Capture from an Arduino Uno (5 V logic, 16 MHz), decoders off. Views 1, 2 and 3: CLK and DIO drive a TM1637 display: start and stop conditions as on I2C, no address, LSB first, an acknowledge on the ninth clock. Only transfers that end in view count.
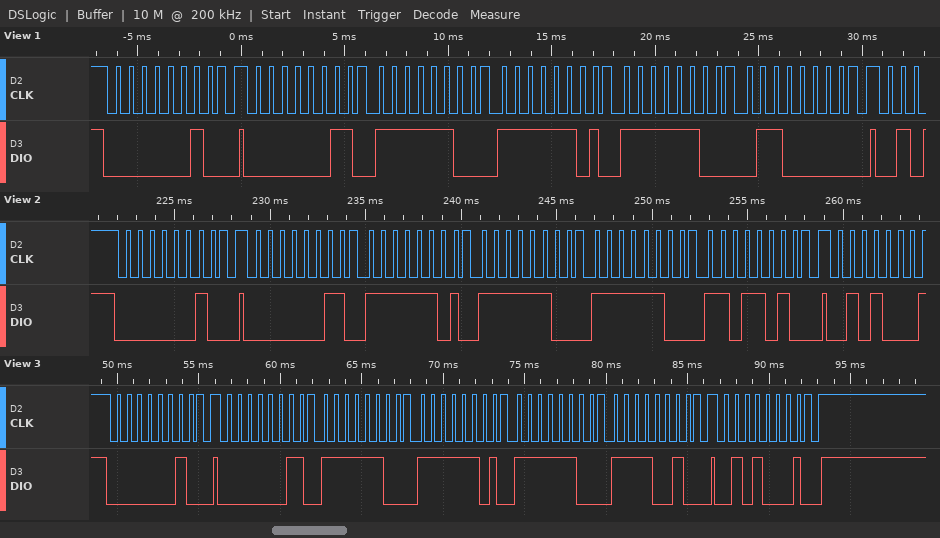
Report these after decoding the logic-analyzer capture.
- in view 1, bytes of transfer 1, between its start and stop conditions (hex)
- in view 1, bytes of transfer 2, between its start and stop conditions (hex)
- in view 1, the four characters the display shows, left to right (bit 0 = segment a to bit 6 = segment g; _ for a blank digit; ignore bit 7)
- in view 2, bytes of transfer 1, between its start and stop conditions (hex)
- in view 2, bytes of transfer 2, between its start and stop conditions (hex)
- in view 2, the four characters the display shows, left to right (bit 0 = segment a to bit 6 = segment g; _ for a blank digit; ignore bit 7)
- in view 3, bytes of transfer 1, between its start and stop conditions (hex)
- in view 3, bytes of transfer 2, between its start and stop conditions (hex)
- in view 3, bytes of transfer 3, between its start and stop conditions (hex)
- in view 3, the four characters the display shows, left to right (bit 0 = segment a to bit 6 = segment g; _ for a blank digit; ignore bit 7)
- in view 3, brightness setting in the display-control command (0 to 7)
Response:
40
C0 3F BF 3F 06
0001
40
C0 BF 3F 3F 5B
0002
40
C0 3F BF 3F 4F
8A
0003
2
